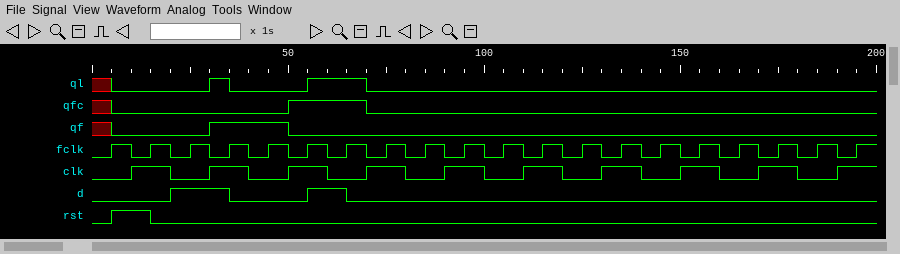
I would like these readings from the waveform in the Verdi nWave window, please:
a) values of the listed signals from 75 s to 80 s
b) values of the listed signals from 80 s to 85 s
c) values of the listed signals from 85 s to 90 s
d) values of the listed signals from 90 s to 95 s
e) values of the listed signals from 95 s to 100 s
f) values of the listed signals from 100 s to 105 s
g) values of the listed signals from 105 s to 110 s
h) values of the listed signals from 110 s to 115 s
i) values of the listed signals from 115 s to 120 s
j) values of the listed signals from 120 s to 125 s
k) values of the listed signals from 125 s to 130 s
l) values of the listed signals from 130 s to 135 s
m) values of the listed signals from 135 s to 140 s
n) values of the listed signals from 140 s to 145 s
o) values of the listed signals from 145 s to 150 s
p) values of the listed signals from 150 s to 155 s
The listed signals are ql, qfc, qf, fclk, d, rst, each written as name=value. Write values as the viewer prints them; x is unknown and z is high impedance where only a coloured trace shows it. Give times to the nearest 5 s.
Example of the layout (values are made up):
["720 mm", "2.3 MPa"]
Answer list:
["ql=0, qfc=0, qf=0, fclk=1, d=0, rst=0", "ql=0, qfc=0, qf=0, fclk=0, d=0, rst=0", "ql=0, qfc=0, qf=0, fclk=1, d=0, rst=0", "ql=0, qfc=0, qf=0, fclk=0, d=0, rst=0", "ql=0, qfc=0, qf=0, fclk=1, d=0, rst=0", "ql=0, qfc=0, qf=0, fclk=0, d=0, rst=0", "ql=0, qfc=0, qf=0, fclk=1, d=0, rst=0", "ql=0, qfc=0, qf=0, fclk=0, d=0, rst=0", "ql=0, qfc=0, qf=0, fclk=1, d=0, rst=0", "ql=0, qfc=0, qf=0, fclk=0, d=0, rst=0", "ql=0, qfc=0, qf=0, fclk=1, d=0, rst=0", "ql=0, qfc=0, qf=0, fclk=0, d=0, rst=0", "ql=0, qfc=0, qf=0, fclk=1, d=0, rst=0", "ql=0, qfc=0, qf=0, fclk=0, d=0, rst=0", "ql=0, qfc=0, qf=0, fclk=1, d=0, rst=0", "ql=0, qfc=0, qf=0, fclk=0, d=0, rst=0"]
